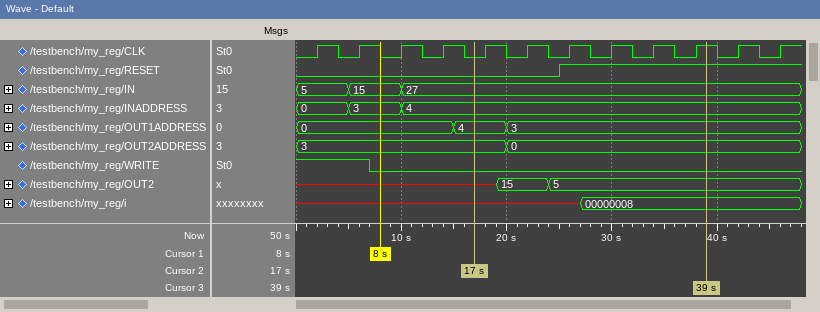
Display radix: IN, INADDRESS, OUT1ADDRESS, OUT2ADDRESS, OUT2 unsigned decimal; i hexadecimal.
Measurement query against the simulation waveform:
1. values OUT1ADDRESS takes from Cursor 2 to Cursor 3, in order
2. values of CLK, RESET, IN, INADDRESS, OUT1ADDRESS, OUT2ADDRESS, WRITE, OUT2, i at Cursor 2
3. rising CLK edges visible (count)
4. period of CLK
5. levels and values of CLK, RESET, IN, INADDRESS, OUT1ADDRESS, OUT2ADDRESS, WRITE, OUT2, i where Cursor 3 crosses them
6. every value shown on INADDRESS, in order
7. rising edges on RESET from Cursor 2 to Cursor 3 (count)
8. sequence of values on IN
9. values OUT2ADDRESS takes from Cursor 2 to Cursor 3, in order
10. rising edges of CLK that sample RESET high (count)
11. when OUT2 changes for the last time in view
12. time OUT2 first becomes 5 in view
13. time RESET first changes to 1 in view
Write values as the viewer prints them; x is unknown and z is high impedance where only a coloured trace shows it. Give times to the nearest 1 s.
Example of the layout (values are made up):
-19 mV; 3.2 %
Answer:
4, 3; CLK=0, RESET=0, IN=27, INADDRESS=4, OUT1ADDRESS=4, OUT2ADDRESS=3, WRITE=0, OUT2=x, i=x; 12; 4 s; CLK=1, RESET=1, IN=27, INADDRESS=4, OUT1ADDRESS=3, OUT2ADDRESS=0, WRITE=0, OUT2=5, i=00000008; 0, 3, 4; 1; 5, 15, 27; 3, 0; 6; 24 s; 24 s; 25 s
